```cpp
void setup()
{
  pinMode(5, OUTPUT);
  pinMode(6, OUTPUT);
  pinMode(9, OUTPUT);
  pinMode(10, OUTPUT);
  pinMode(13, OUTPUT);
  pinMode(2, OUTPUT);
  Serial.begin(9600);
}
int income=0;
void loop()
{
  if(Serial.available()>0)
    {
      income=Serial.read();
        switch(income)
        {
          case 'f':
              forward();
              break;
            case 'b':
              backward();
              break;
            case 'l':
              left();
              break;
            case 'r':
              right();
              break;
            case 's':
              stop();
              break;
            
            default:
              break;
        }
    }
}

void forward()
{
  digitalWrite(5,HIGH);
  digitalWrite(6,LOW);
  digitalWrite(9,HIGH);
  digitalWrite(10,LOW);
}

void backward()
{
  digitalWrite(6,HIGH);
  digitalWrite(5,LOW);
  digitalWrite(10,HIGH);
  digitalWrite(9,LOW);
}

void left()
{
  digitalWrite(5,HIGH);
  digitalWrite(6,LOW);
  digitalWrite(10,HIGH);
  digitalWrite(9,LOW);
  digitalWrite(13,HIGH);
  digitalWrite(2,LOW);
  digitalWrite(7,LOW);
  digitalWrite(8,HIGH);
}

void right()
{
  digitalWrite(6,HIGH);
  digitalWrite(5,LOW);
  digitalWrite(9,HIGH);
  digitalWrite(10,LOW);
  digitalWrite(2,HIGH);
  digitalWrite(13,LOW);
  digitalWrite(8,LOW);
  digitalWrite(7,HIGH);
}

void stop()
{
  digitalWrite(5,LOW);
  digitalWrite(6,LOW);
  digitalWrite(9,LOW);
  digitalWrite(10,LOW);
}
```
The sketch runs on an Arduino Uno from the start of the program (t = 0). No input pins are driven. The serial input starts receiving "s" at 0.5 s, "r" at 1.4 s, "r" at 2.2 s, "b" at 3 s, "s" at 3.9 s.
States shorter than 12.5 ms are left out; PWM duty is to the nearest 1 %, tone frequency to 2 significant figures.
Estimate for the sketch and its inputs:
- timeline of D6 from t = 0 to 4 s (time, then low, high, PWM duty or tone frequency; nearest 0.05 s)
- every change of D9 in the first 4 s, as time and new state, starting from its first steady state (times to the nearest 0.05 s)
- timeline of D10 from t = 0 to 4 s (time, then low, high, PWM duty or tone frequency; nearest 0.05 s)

0 s low; 1.4 s high; 3.9 s low
0 s low; 1.4 s high; 3 s low
0 s low; 3 s high; 3.9 s low
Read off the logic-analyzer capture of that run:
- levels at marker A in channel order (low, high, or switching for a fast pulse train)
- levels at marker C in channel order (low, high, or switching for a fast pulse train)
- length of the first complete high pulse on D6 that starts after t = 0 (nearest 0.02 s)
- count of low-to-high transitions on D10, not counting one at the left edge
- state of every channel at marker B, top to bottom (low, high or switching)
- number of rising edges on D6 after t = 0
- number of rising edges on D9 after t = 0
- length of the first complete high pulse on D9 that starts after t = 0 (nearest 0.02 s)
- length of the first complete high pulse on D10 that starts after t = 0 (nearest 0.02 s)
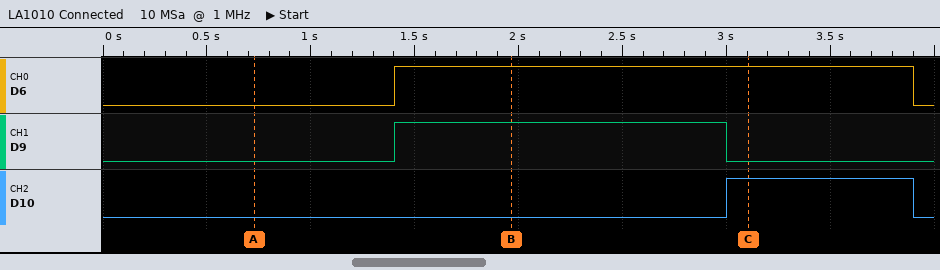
D6 low, D9 low, D10 low
D6 high, D9 low, D10 high
2.50 s
1
D6 high, D9 high, D10 low
1
1
1.60 s
0.90 s
